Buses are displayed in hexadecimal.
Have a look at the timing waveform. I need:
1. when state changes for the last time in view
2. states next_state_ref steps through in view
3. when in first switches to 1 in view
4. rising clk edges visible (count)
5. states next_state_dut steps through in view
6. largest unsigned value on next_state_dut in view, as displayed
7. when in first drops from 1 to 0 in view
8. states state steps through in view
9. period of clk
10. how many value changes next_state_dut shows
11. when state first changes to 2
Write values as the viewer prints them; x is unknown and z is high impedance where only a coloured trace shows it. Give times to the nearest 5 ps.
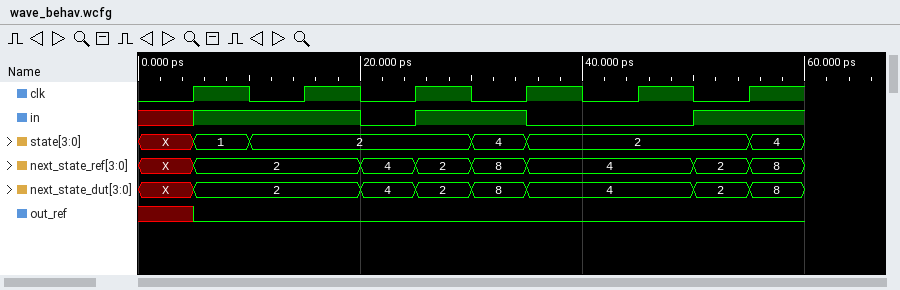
55 ps
X, 2, 4, 2, 8, 4, 2, 8
5 ps
6
X, 2, 4, 2, 8, 4, 2, 8
8
20 ps
X, 1, 2, 4, 2, 4
10 ps
7
10 ps
